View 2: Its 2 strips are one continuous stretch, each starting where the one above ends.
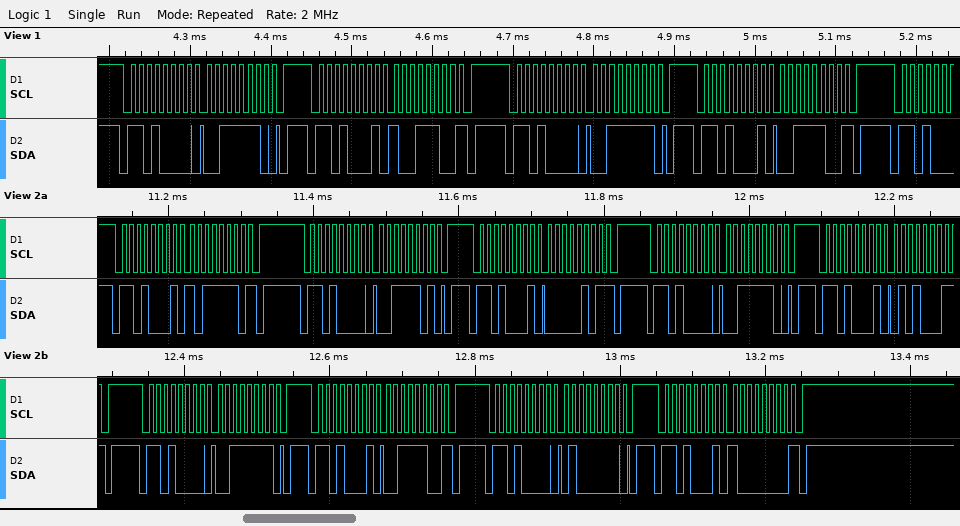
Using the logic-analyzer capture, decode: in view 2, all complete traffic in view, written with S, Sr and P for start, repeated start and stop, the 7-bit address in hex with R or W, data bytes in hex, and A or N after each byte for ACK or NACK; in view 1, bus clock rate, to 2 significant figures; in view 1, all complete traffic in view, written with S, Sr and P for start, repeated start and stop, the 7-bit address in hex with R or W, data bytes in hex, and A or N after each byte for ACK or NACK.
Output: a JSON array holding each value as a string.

["S 68R A BE N P S 68W A 3D A P S 68R A 05 N P S 68W A 3E A P S 68R A 51 N P S 68W A 3F A P S 68R A 3C N P S 68W A 40 A P S 68R A 80 N P", "100 kHz", "S 68W A 3E A P S 68R A 9C N P S 68W A 3F A P S 68R A 3C N P"]
